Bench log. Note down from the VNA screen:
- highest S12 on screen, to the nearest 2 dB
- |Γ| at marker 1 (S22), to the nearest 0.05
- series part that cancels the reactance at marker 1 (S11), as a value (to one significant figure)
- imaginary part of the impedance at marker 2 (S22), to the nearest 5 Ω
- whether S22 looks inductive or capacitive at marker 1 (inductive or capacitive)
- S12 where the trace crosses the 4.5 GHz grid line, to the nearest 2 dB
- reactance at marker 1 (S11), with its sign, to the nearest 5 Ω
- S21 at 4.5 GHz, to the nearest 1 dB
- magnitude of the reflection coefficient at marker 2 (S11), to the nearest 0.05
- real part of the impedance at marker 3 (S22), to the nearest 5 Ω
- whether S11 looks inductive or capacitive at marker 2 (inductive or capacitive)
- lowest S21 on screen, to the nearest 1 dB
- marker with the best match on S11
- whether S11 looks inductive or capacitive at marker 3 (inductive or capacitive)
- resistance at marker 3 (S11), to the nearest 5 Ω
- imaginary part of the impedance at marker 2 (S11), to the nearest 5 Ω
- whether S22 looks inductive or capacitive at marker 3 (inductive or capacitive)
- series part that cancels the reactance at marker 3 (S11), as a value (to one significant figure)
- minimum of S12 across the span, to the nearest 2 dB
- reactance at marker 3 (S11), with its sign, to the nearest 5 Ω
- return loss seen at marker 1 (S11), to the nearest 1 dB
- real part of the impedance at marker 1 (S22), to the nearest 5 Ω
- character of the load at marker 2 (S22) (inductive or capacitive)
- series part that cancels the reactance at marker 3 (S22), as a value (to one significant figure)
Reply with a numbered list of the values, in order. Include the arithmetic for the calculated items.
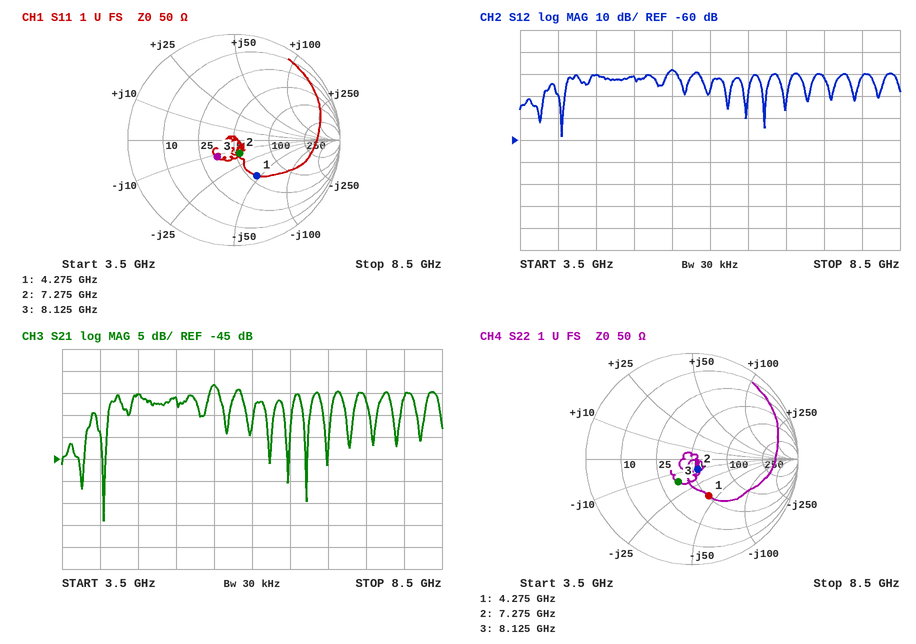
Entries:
1. -28 dB
2. 0.40
3. L = 45 Ω/(2π × 4.275 GHz) ≈ 2 nH
4. -10 Ω
5. capacitive
6. -30 dB
7. -45 Ω
8. -30 dB
9. 0.15
10. 35 Ω
11. capacitive
12. -59 dB
13. marker 2
14. capacitive
15. 35 Ω
16. -15 Ω
17. capacitive
18. L = 10 Ω/(2π × 8.125 GHz) ≈ 196 pH, so 200 pH to one significant figure
19. -58 dB
20. -10 Ω
21. 8 dB
22. 50 Ω
23. capacitive
24. L = 15 Ω/(2π × 8.125 GHz) ≈ 294 pH, so 300 pH to one significant figure
